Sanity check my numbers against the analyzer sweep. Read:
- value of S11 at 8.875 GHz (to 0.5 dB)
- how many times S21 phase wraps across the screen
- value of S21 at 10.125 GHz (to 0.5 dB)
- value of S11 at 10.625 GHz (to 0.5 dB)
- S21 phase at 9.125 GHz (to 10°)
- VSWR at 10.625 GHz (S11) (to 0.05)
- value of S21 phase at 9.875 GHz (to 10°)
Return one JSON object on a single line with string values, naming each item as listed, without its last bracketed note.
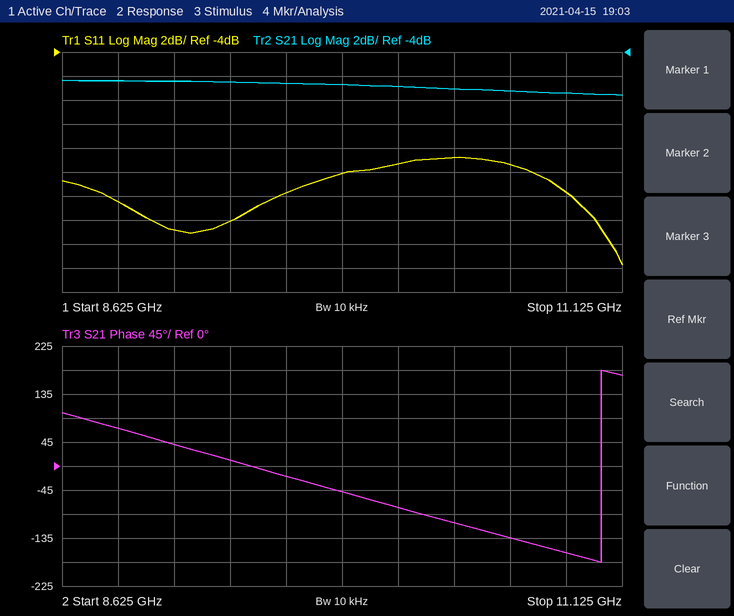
{"value of S11 at 8.875 GHz": "-16.5 dB", "how many times S21 phase wraps across the screen": "1", "value of S21 at 10.125 GHz": "-7.0 dB", "value of S11 at 10.625 GHz": "-13.5 dB", "S21 phase at 9.125 GHz": "40°", "VSWR at 10.625 GHz (S11)": "1.55", "value of S21 phase at 9.875 GHz": "-50°"}
